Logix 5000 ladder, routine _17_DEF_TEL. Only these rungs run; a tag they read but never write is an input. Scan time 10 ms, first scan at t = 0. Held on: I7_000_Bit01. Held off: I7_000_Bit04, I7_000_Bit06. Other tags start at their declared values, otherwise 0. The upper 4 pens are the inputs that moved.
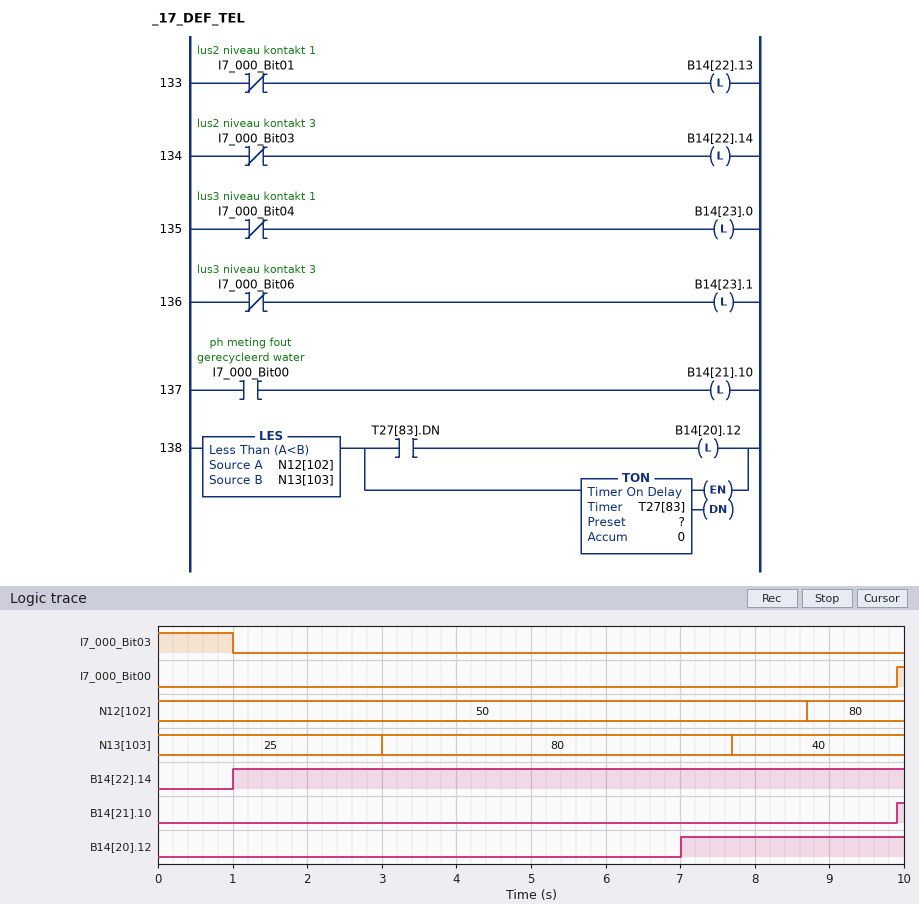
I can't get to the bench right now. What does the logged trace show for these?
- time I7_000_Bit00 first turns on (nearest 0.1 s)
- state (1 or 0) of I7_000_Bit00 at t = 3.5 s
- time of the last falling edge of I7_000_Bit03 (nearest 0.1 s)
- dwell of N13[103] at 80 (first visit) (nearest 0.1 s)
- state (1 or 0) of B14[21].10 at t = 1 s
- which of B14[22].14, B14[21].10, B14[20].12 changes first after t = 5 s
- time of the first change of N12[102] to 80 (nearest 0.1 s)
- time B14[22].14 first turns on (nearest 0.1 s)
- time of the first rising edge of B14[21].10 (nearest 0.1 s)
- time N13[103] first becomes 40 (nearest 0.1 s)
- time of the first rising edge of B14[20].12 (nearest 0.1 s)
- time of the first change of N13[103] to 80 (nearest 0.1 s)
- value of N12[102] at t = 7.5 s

9.9 s
0
1.0 s
4.7 s
0
B14[20].12
8.7 s
1.0 s
9.9 s
7.7 s
7.0 s
3.0 s
50
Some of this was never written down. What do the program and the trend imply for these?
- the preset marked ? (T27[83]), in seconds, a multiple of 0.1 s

4.0 s
